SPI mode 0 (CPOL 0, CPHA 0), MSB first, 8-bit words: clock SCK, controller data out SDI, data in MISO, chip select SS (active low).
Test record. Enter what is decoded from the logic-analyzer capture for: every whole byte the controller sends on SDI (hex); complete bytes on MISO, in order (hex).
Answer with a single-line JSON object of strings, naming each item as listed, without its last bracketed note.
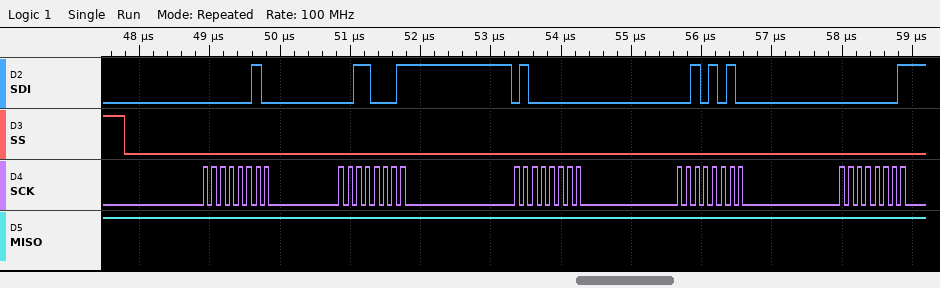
{"every whole byte the controller sends on SDI": "02 31 40 2A 01", "complete bytes on MISO, in order": "FF FF FF FF FF"}
